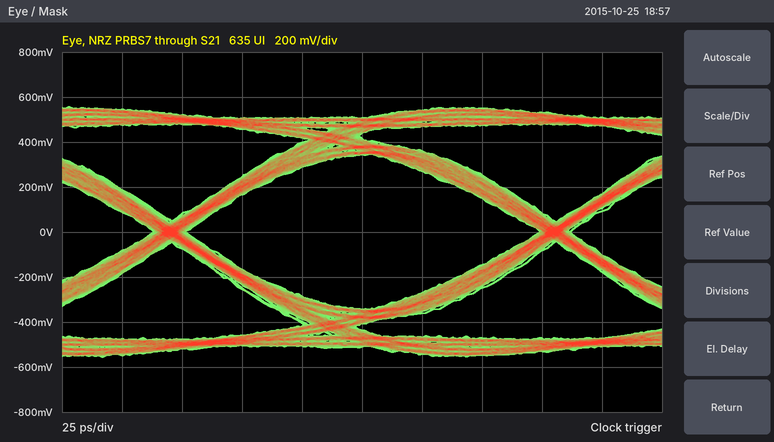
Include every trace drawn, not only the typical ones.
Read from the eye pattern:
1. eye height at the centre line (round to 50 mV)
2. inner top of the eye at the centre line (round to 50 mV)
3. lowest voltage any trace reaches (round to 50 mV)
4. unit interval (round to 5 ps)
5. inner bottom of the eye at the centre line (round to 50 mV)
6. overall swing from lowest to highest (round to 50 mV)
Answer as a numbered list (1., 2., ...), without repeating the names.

1. 700 mV
2. 350 mV
3. -550 mV
4. 160 ps
5. -350 mV
6. 1.10 V
